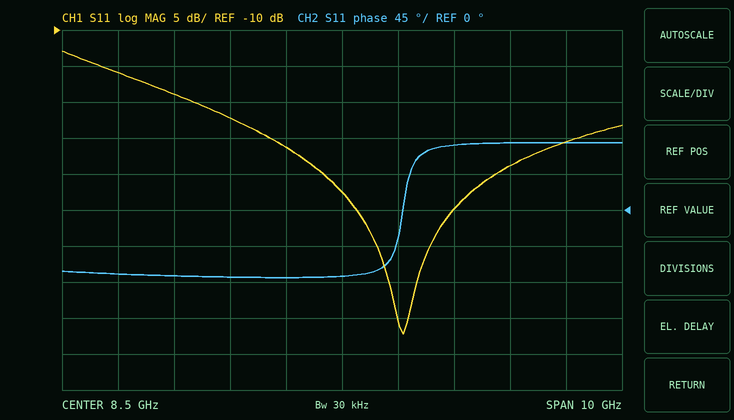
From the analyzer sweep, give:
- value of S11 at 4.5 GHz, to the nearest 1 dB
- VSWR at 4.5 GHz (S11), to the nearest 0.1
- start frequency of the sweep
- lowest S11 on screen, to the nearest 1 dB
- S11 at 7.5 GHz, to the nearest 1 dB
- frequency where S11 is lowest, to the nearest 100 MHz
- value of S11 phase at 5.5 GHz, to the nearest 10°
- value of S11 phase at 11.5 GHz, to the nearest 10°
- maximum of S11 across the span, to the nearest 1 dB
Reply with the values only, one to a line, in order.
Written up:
-16 dB
1.4
3.5 GHz
-52 dB
-26 dB
9.6 GHz
-80°
80°
-13 dB
